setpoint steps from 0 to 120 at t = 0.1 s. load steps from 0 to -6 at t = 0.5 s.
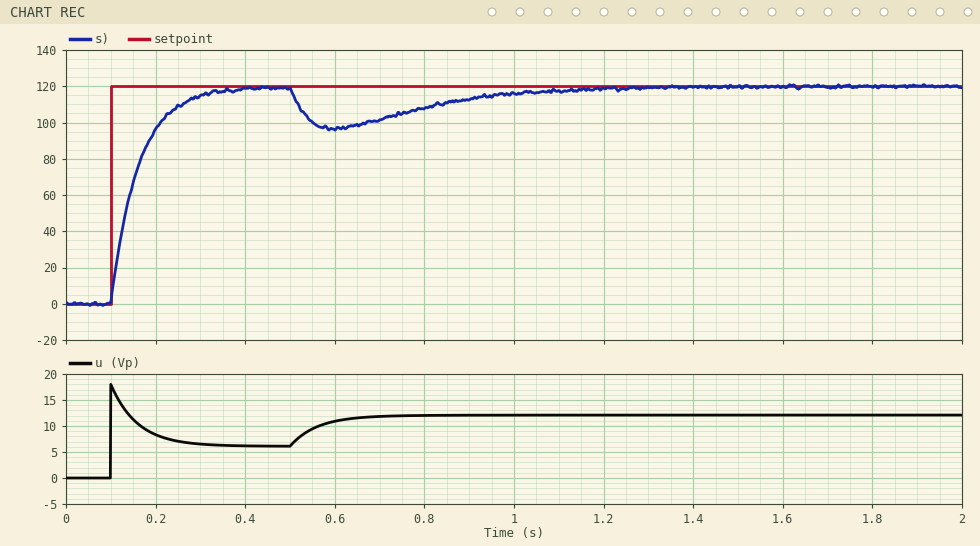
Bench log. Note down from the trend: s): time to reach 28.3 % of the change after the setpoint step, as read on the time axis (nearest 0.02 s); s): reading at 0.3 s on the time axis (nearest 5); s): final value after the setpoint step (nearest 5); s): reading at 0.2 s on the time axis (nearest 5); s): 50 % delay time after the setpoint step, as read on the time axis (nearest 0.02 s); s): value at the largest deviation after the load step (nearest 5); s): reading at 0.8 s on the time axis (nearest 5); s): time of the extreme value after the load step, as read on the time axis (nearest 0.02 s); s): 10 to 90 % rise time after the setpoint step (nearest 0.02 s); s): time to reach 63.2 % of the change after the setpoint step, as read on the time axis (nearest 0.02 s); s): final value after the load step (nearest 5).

0.12 s
115
120
95
0.14 s
95
110
0.60 s
0.14 s
0.16 s
120
